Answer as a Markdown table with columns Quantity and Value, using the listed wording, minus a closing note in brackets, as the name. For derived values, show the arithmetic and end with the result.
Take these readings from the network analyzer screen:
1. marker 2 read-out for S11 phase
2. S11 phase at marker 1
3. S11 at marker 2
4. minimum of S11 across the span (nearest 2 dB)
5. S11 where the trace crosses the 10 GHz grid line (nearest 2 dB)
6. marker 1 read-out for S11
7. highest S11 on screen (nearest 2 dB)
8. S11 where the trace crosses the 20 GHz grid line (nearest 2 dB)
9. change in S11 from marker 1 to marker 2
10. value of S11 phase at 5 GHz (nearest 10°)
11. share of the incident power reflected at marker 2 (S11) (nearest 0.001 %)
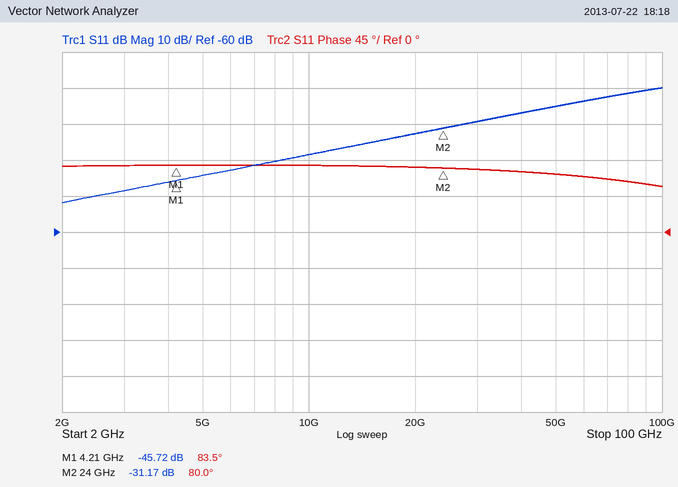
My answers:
| Quantity | Value |
|---|---|
| marker 2 read-out for S11 phase | 80.0° |
| S11 phase at marker 1 | 83.5° |
| S11 at marker 2 | -31.17 dB |
| minimum of S11 across the span | -52 dB |
| S11 where the trace crosses the 10 GHz grid line | -38 dB |
| marker 1 read-out for S11 | -45.72 dB |
| highest S11 on screen | -20 dB |
| S11 where the trace crosses the 20 GHz grid line | -32 dB |
| change in S11 from marker 1 to marker 2 | -31.17 − (-45.72) = 14.55 dB |
| value of S11 phase at 5 GHz | 80° |
| share of the incident power reflected at marker 2 (S11) | 10^(-31.17/10) ≈ 0.076 % |
